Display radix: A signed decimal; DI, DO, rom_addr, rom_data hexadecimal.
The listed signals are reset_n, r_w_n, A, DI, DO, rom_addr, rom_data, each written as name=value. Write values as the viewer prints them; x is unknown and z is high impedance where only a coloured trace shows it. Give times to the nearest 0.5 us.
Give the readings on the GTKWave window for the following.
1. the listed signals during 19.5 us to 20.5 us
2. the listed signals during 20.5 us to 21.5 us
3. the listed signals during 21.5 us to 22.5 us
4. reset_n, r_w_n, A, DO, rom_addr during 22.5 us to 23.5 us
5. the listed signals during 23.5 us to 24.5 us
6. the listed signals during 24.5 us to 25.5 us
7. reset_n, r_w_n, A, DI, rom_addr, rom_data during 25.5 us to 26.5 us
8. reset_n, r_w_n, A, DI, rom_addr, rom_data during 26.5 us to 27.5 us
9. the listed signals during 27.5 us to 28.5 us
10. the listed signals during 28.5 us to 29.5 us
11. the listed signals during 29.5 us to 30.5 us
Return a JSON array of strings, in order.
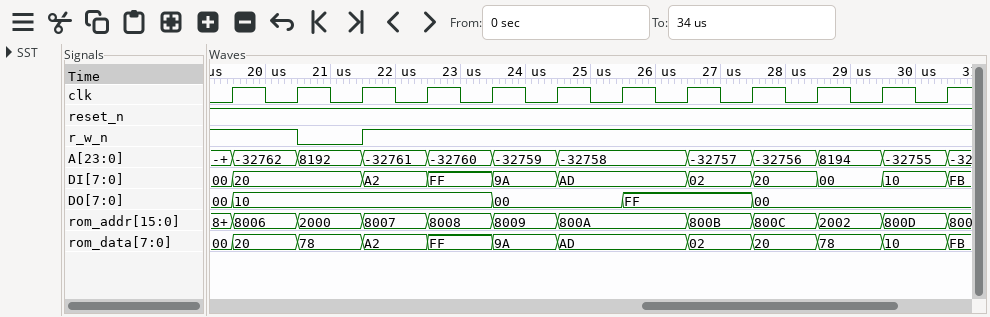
["reset_n=1, r_w_n=1, A=-32762, DI=20, DO=10, rom_addr=8006, rom_data=20", "reset_n=1, r_w_n=0, A=8192, DI=20, DO=10, rom_addr=2000, rom_data=78", "reset_n=1, r_w_n=1, A=-32761, DI=A2, DO=10, rom_addr=8007, rom_data=A2", "reset_n=1, r_w_n=1, A=-32760, DO=10, rom_addr=8008", "reset_n=1, r_w_n=1, A=-32759, DI=9A, DO=00, rom_addr=8009, rom_data=9A", "reset_n=1, r_w_n=1, A=-32758, DI=AD, DO=00, rom_addr=800A, rom_data=AD", "reset_n=1, r_w_n=1, A=-32758, DI=AD, rom_addr=800A, rom_data=AD", "reset_n=1, r_w_n=1, A=-32757, DI=02, rom_addr=800B, rom_data=02", "reset_n=1, r_w_n=1, A=-32756, DI=20, DO=00, rom_addr=800C, rom_data=20", "reset_n=1, r_w_n=1, A=8194, DI=00, DO=00, rom_addr=2002, rom_data=78", "reset_n=1, r_w_n=1, A=-32755, DI=10, DO=00, rom_addr=800D, rom_data=10"]
